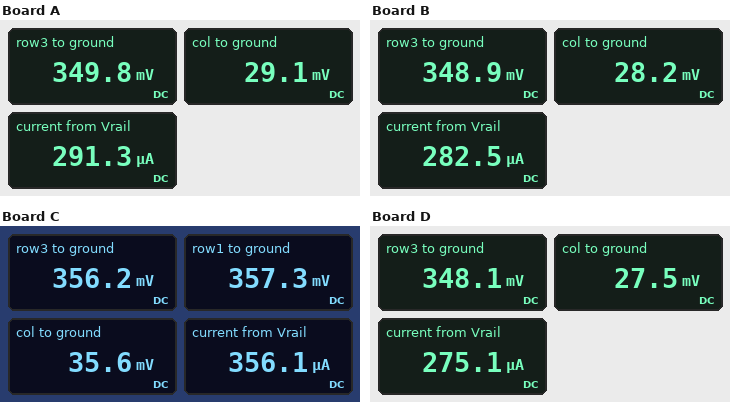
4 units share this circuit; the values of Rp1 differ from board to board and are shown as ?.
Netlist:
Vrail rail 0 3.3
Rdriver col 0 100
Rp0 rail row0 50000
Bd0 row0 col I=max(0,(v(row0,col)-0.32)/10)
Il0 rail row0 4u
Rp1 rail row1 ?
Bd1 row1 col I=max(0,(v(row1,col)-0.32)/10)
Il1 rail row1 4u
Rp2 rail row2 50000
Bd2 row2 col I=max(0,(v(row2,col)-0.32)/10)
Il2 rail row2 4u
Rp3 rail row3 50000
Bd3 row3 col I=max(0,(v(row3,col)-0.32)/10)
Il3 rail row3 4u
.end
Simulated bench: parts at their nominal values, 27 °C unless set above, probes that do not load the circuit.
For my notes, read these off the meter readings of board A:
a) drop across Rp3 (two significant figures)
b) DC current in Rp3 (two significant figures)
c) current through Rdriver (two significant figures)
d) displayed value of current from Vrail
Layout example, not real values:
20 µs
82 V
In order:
3.0 V
59 µA
290 µA
291.3 µA
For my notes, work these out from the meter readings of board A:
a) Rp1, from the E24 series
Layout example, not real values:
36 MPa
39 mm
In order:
30 kΩ
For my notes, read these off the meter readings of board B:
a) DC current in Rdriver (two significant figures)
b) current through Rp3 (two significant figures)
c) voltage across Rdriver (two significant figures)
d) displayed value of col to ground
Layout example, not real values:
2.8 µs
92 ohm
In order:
280 µA
59 µA
28 mV
28.2 mV
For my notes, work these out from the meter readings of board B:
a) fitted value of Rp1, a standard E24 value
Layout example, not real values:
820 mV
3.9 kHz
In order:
33 kΩ
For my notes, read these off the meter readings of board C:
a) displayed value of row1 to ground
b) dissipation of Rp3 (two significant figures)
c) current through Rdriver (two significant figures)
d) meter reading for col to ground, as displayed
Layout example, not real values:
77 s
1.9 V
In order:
357.3 mV
170 µW
360 µA
35.6 mV
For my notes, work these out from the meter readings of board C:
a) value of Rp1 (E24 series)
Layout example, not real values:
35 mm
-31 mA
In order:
18 kΩ
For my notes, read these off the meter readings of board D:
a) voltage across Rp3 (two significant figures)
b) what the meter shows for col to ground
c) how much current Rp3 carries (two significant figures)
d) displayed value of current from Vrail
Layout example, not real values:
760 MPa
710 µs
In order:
3.0 V
27.5 mV
59 µA
275.1 µA
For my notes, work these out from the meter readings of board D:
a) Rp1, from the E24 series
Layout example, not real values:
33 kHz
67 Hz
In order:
36 kΩ
